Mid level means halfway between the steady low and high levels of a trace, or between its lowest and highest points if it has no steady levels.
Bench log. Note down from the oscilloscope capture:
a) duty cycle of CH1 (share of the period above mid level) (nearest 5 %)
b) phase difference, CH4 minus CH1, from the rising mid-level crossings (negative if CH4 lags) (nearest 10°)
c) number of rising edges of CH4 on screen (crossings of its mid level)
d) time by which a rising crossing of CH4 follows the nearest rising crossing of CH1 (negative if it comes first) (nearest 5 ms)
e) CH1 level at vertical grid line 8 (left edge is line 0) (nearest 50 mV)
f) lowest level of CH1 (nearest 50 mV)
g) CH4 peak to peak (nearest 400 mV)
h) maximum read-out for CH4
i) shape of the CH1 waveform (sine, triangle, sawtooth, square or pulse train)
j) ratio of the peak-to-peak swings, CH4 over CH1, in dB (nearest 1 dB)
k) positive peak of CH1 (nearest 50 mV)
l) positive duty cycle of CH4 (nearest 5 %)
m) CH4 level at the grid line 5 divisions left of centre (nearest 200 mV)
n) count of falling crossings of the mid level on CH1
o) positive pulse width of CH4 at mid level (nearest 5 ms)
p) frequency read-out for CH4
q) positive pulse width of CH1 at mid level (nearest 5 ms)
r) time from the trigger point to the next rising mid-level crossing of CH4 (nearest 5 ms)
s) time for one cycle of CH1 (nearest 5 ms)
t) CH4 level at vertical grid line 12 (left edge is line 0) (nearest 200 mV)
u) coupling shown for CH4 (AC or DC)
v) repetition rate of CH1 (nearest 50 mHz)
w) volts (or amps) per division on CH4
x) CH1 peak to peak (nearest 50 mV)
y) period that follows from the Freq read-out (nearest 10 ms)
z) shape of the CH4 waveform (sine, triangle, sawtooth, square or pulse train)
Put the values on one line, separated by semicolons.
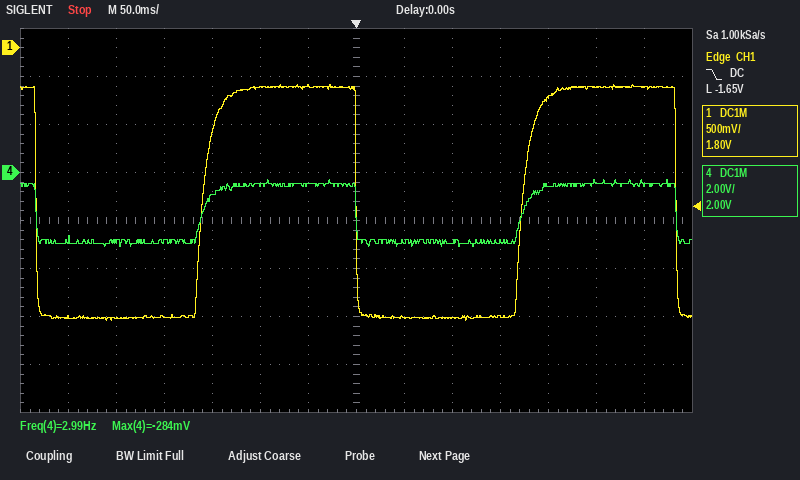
50 %; 0°; 2; 0 ms; -2.80 V; -2.85 V; 2.8 V; -284 mV; square; 1 dB; -400 mV; 50 %; -2.8 V; 3; 160 ms; 2.99 Hz; 160 ms; 175 ms; 335 ms; -400 mV; DC; 3.00 Hz; 2 V; 2.45 V; 330 ms; square
